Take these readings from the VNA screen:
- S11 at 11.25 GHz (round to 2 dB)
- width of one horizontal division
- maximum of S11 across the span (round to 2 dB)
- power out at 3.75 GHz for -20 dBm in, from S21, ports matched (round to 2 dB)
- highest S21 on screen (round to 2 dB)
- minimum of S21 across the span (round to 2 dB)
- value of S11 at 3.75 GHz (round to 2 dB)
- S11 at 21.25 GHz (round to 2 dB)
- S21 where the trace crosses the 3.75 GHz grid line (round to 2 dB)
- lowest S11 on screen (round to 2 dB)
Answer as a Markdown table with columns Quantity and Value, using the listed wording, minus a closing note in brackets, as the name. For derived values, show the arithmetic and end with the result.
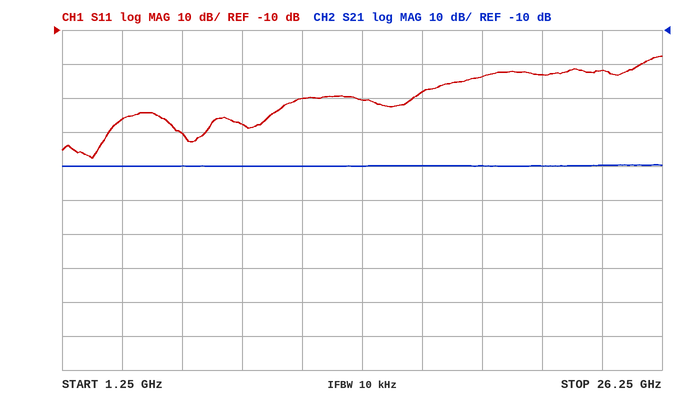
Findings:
| Quantity | Value |
|---|---|
| S11 at 11.25 GHz | -30 dB |
| width of one horizontal division | 2.5 GHz |
| maximum of S11 across the span | -18 dB |
| power out at 3.75 GHz for -20 dBm in, from S21, ports matched | -20 dBm + (-50 dB) = -70 dBm |
| highest S21 on screen | -50 dB |
| minimum of S21 across the span | -50 dB |
| value of S11 at 3.75 GHz | -36 dB |
| S11 at 21.25 GHz | -24 dB |
| S21 where the trace crosses the 3.75 GHz grid line | -50 dB |
| lowest S11 on screen | -48 dB |
